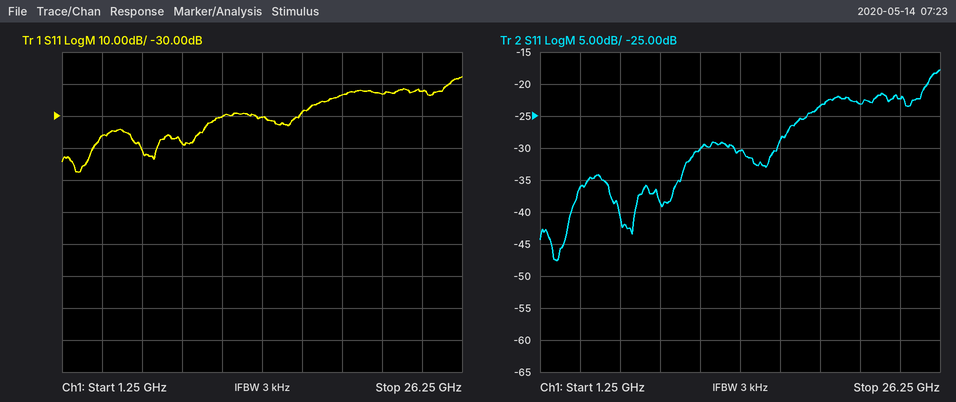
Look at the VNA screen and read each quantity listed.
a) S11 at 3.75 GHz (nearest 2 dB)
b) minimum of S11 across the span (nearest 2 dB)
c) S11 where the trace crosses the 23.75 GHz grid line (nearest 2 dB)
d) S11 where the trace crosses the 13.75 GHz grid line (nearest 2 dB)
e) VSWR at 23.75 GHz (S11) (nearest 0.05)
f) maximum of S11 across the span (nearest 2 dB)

-36 dB
-48 dB
-22 dB
-30 dB
1.15
-18 dB
